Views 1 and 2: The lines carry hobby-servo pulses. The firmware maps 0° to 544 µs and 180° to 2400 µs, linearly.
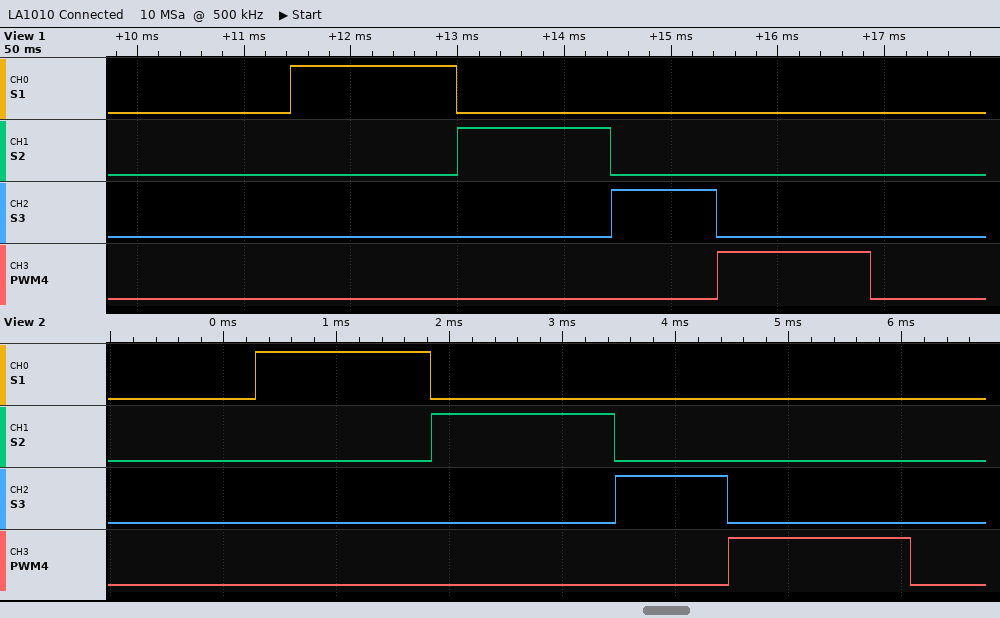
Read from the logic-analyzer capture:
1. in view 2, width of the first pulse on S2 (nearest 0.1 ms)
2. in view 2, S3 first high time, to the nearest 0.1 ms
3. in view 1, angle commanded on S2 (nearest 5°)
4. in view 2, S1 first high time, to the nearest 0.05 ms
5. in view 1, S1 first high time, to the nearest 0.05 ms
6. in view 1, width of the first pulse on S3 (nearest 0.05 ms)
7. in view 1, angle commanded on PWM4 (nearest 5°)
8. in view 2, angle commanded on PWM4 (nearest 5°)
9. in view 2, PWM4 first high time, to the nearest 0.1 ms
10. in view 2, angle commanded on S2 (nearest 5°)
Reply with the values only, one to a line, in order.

1.6 ms
1.0 ms
85°
1.55 ms
1.55 ms
1.00 ms
85°
105°
1.6 ms
105°
